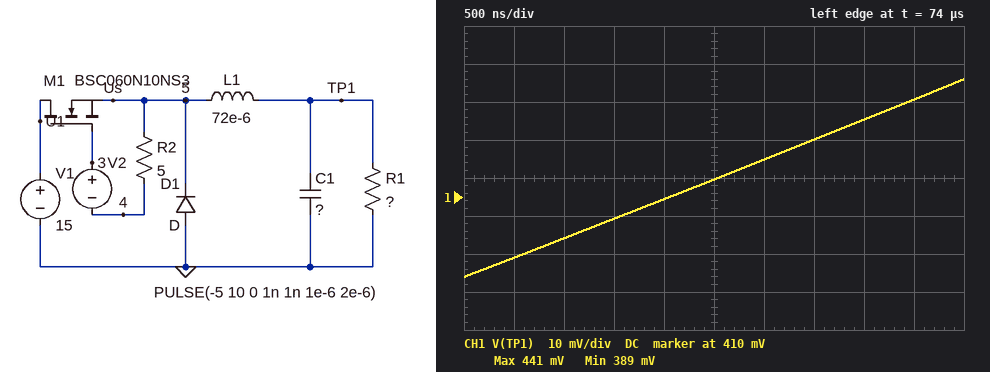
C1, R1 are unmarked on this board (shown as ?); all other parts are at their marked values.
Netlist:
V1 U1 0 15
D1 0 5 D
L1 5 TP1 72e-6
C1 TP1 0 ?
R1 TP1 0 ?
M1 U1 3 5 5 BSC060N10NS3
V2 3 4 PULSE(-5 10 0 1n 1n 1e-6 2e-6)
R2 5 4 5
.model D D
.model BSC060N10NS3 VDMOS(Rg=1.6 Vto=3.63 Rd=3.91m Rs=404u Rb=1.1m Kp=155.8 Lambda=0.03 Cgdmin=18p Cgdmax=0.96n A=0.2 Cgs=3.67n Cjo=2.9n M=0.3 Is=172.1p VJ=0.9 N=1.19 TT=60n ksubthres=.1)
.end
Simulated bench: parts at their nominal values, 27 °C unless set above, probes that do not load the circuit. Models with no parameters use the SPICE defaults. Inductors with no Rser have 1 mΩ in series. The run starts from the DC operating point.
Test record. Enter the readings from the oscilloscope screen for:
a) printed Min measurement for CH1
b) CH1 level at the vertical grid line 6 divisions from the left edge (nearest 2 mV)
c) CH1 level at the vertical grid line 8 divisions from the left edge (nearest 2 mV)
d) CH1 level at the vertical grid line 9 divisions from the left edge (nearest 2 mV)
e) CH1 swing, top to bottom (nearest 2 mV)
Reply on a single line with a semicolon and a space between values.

389 mV; 420 mV; 430 mV; 436 mV; 52 mV
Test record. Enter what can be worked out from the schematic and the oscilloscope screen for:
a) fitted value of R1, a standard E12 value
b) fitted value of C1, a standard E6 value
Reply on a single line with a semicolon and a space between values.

1.2 Ω; 680 µF
